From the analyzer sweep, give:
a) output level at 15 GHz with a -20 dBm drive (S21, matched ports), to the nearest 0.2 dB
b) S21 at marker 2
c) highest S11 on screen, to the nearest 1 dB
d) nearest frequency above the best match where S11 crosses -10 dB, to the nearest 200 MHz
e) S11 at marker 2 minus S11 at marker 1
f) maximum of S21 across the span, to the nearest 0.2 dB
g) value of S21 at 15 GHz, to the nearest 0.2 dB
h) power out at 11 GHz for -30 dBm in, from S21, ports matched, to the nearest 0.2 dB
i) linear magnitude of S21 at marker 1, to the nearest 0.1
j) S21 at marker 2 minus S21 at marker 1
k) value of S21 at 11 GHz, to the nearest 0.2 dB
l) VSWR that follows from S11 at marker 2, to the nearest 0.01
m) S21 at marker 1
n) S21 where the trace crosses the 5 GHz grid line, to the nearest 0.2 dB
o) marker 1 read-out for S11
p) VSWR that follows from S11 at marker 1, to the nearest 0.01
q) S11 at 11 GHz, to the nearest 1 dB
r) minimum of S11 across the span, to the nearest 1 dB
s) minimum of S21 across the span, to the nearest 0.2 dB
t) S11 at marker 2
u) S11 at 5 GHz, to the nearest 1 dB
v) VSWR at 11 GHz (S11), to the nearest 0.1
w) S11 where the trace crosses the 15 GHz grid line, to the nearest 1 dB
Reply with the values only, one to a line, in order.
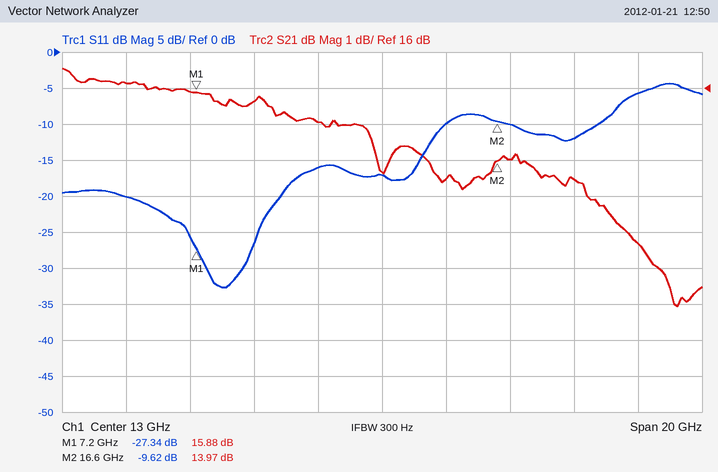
-6.6 dBm
13.97 dB
-4 dB
15.0 GHz
17.72 dB
16.6 dB
13.4 dB
-15.0 dBm
6.2
-1.91 dB
15.0 dB
1.99
15.88 dB
16.2 dB
-27.34 dB
1.09
-16 dB
-33 dB
10.0 dB
-9.62 dB
-20 dB
1.4
-10 dB
